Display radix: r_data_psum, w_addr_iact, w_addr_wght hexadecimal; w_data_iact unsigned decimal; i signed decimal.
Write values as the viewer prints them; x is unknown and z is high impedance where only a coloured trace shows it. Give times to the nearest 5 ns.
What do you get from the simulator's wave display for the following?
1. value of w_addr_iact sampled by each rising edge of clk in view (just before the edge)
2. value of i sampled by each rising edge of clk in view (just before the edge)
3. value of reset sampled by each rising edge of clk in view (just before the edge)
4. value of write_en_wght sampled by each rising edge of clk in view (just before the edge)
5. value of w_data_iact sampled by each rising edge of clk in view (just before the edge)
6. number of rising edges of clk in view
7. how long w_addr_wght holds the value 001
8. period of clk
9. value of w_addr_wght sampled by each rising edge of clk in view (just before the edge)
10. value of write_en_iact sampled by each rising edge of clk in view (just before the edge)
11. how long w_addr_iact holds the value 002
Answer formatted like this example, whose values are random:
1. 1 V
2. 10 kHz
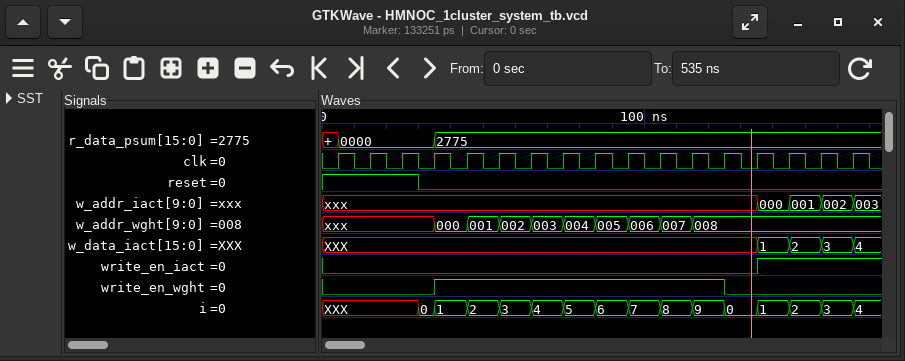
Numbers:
1. xxx, xxx, xxx, xxx, xxx, xxx, xxx, xxx, xxx, xxx, xxx, xxx, xxx, xxx, 000, 001, 002
2. XXX, XXX, XXX, 0, 1, 2, 3, 4, 5, 6, 7, 8, 9, 0, 1, 2, 3
3. 1 1 1 0 0 0 0 0 0 0 0 0 0 0 0 0 0
4. 0 0 0 0 1 1 1 1 1 1 1 1 1 0 0 0 0
5. XXX, XXX, XXX, XXX, XXX, XXX, XXX, XXX, XXX, XXX, XXX, XXX, XXX, XXX, 1, 2, 3
6. 17
7. 10 ns
8. 10 ns
9. xxx, xxx, xxx, xxx, 000, 001, 002, 003, 004, 005, 006, 007, 008, 008, 008, 008, 008
10. 0 0 0 0 0 0 0 0 0 0 0 0 0 0 1 1 1
11. 10 ns
